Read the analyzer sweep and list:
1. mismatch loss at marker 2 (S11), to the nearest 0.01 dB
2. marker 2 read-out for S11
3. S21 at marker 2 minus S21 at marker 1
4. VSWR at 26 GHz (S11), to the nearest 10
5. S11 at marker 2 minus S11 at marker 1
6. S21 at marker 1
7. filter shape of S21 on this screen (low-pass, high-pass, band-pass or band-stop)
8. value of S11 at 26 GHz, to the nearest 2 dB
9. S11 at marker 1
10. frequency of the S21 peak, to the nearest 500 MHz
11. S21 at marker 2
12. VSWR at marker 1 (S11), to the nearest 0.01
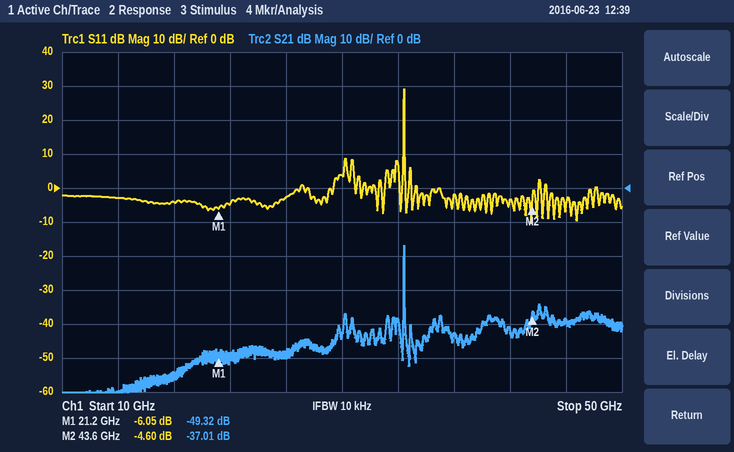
1.85 dB
-4.60 dB
12.31 dB
10
1.45 dB
-49.32 dB
band-pass
-2 dB
-6.05 dB
34.5 GHz
-37.01 dB
2.99
